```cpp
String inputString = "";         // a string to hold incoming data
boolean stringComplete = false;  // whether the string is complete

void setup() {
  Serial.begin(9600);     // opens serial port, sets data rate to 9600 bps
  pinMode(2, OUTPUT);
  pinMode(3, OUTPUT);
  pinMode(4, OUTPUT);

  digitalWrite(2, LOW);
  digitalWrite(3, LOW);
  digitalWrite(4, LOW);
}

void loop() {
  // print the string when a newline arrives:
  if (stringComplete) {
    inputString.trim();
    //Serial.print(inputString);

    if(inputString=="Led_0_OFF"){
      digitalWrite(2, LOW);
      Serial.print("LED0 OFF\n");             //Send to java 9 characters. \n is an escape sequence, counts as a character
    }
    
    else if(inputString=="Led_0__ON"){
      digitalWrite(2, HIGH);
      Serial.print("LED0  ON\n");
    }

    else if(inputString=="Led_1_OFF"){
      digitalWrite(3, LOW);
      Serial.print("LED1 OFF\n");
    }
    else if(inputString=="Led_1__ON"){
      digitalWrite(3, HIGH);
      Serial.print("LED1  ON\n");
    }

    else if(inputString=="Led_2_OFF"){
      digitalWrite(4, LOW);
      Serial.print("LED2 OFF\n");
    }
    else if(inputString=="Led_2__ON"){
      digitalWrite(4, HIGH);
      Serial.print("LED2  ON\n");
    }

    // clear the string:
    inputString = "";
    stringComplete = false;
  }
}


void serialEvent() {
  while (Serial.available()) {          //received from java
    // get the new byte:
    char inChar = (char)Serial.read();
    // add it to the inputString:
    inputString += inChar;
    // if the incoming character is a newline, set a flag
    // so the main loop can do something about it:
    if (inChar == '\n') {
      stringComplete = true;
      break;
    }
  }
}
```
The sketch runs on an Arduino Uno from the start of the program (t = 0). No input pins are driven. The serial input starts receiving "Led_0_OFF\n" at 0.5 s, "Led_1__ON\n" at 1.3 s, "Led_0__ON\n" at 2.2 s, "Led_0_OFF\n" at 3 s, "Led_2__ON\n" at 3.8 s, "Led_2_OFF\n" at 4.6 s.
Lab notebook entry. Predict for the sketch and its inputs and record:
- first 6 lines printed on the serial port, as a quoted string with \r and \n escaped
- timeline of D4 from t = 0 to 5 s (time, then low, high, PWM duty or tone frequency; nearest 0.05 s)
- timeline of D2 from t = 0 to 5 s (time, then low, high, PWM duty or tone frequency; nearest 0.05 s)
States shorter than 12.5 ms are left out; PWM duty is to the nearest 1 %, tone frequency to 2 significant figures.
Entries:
"LED0 OFF\nLED1  ON\nLED0  ON\nLED0 OFF\nLED2  ON\nLED2 OFF\n"
0 s low; 3.8 s high; 4.6 s low
0 s low; 2.2 s high; 3 s low
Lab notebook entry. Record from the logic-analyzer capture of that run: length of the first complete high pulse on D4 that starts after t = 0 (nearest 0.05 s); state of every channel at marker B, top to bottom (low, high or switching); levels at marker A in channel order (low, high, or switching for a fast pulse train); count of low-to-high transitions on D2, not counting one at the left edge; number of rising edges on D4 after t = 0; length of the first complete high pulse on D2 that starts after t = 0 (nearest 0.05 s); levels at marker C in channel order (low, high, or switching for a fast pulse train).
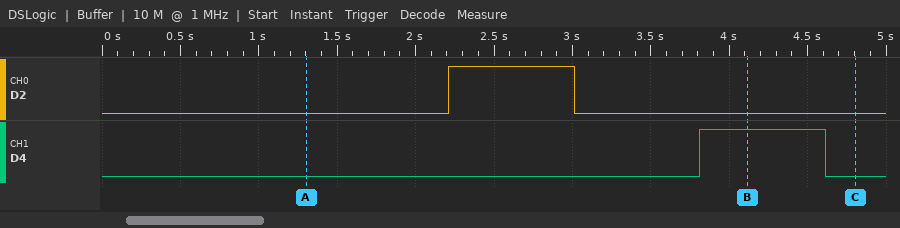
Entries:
0.80 s
D2 low, D4 high
D2 low, D4 low
1
1
0.80 s
D2 low, D4 low
